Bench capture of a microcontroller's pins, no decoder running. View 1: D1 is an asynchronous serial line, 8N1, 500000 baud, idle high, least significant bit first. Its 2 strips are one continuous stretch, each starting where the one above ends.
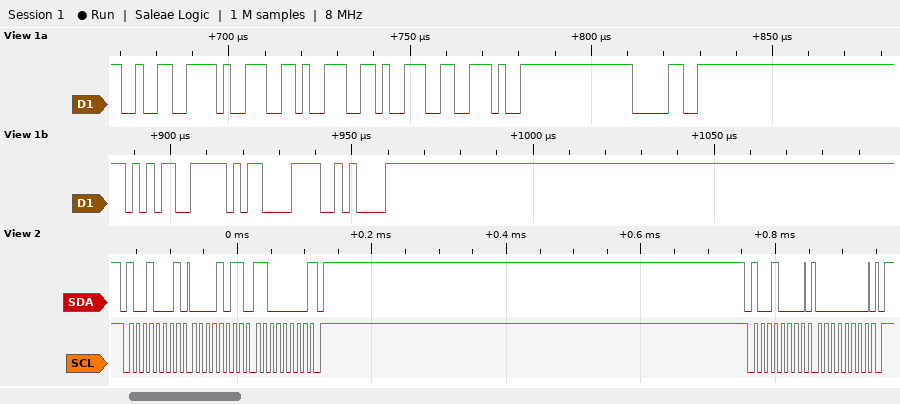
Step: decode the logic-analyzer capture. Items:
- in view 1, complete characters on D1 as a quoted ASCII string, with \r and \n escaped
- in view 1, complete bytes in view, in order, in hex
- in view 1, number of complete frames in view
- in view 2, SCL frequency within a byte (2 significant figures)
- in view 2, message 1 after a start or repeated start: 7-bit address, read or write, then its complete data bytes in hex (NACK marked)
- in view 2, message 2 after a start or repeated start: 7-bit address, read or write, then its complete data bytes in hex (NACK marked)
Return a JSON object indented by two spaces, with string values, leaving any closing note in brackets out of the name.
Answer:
{
  "in view 1, complete characters on D1 as a quoted ASCII string, with \\r and \\n escaped": "\"2999.05\\r\\n\"",
  "in view 1, complete bytes in view, in order, in hex": "32 39 39 39 2E 30 35 0D 0A",
  "in view 1, number of complete frames in view": "9",
  "in view 2, SCL frequency within a byte": "100 kHz",
  "in view 2, message 1 after a start or repeated start: 7-bit address, read or write, then its complete data bytes in hex": "0x48 read: 0B C0 NACK",
  "in view 2, message 2 after a start or repeated start: 7-bit address, read or write, then its complete data bytes in hex": "0x48 write: 00"
}
